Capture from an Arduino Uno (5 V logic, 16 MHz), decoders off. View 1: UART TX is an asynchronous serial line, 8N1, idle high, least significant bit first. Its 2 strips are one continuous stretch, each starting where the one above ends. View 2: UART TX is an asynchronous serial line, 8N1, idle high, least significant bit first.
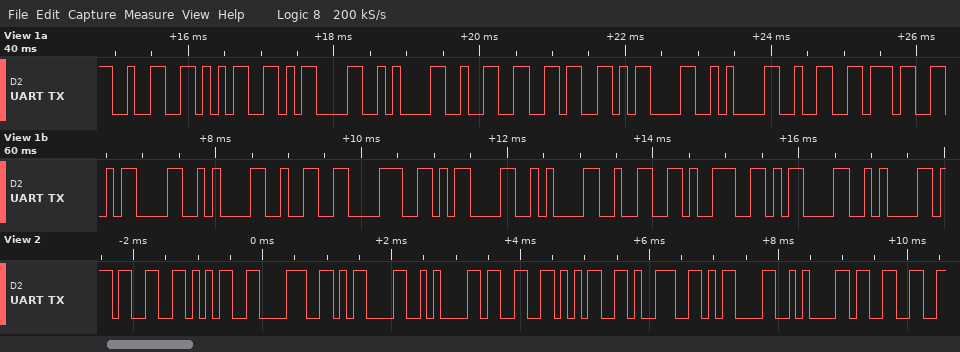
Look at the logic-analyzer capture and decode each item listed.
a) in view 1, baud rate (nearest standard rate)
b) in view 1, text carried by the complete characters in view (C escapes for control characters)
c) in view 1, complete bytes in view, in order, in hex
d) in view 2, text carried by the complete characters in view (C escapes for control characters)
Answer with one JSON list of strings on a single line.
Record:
["9600 baud", "\"25\\r\\n26\\r\\n27\\r\\n28\\r\\n29\\r\\n\"", "32 35 0D 0A 32 36 0D 0A 32 37 0D 0A 32 38 0D 0A 32 39 0D 0A", "\"358\\r\\n359\\r\\n3\""]
